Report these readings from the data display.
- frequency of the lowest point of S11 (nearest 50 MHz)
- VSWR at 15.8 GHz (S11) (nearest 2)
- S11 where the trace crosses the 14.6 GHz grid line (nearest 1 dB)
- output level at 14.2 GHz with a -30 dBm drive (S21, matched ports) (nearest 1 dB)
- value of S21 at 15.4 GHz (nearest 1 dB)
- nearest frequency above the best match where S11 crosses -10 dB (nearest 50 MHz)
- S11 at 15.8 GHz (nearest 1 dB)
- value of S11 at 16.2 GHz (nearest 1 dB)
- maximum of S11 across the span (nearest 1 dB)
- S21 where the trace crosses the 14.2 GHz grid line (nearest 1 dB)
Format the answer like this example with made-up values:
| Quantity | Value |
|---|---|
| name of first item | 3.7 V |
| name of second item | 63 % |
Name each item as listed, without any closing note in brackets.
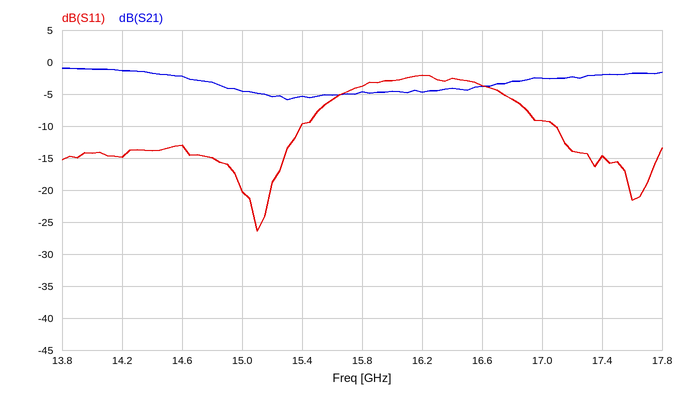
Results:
| Quantity | Value |
|---|---|
| frequency of the lowest point of S11 | 15.10 GHz |
| VSWR at 15.8 GHz (S11) | 4 |
| S11 where the trace crosses the 14.6 GHz grid line | -13 dB |
| output level at 14.2 GHz with a -30 dBm drive (S21, matched ports) | -31 dBm |
| value of S21 at 15.4 GHz | -5 dB |
| nearest frequency above the best match where S11 crosses -10 dB | 15.40 GHz |
| S11 at 15.8 GHz | -4 dB |
| value of S11 at 16.2 GHz | -2 dB |
| maximum of S11 across the span | -2 dB |
| S21 where the trace crosses the 14.2 GHz grid line | -1 dB |
